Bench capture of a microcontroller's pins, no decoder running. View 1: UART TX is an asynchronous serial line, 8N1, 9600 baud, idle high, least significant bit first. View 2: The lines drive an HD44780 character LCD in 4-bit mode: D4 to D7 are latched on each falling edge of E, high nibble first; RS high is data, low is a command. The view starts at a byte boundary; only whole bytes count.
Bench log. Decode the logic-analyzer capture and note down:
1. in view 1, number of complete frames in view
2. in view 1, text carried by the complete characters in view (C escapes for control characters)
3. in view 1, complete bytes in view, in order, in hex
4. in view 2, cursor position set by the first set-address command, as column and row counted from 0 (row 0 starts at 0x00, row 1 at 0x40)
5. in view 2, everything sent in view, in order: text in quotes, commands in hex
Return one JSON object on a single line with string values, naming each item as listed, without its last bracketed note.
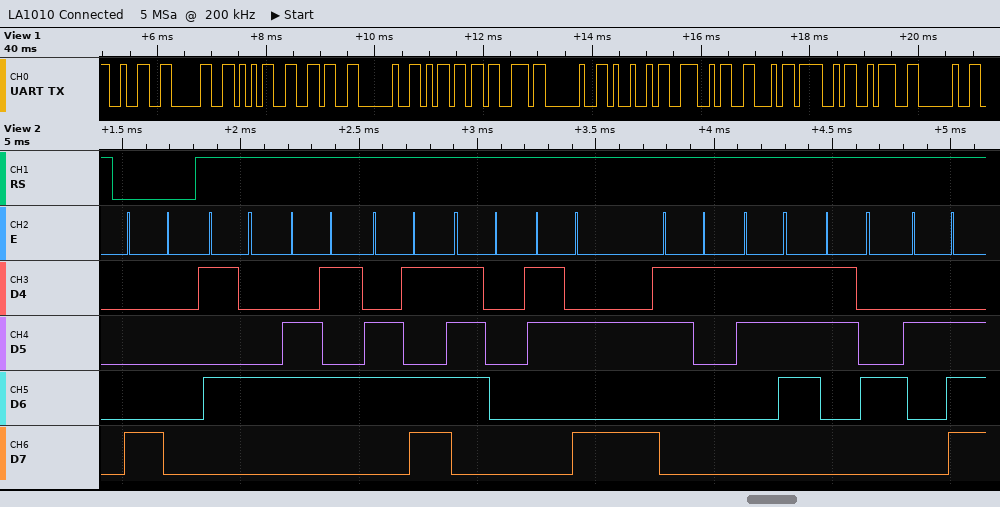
{"in view 1, number of complete frames in view": "14", "in view 1, text carried by the complete characters in view": "\"2056 ms INFO: \"", "in view 1, complete bytes in view, in order, in hex": "32 30 35 36 20 6D 73 20 49 4E 46 4F 3A 20", "in view 2, cursor position set by the first set-address command, as column and row counted from 0": "column 0, row 0", "in view 2, everything sent in view, in order: text in quotes, commands in hex": "0x80 \"Temp:174.\""}
